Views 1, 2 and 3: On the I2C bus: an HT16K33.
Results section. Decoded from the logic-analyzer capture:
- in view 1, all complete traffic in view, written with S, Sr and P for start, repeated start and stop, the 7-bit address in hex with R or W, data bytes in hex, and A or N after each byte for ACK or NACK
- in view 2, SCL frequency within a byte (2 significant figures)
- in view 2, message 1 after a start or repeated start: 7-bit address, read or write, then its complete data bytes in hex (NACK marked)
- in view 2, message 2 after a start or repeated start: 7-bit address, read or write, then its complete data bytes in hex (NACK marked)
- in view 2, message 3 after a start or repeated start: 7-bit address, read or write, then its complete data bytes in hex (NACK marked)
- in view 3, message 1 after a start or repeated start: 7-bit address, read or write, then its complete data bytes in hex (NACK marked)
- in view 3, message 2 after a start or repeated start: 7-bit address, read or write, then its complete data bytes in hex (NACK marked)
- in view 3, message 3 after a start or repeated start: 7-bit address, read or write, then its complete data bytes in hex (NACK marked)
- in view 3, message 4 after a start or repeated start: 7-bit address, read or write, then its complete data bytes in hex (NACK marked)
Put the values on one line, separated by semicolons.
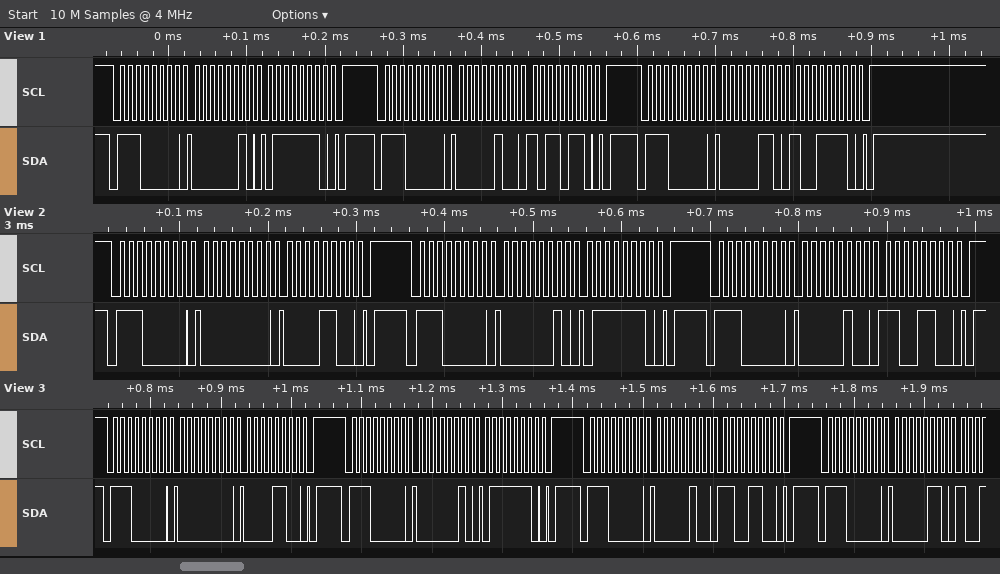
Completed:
S 70W A 02 A 7E A P S 70W A 04 A B6 A P S 70W A 06 A 9E A P; 100 kHz; 0x70 write: 00 0C; 0x70 write: 02 7E; 0x70 write: 04 CC; 0x70 write: 00 0C; 0x70 write: 02 7E; 0x70 write: 04 CC; 0x70 write: 06
